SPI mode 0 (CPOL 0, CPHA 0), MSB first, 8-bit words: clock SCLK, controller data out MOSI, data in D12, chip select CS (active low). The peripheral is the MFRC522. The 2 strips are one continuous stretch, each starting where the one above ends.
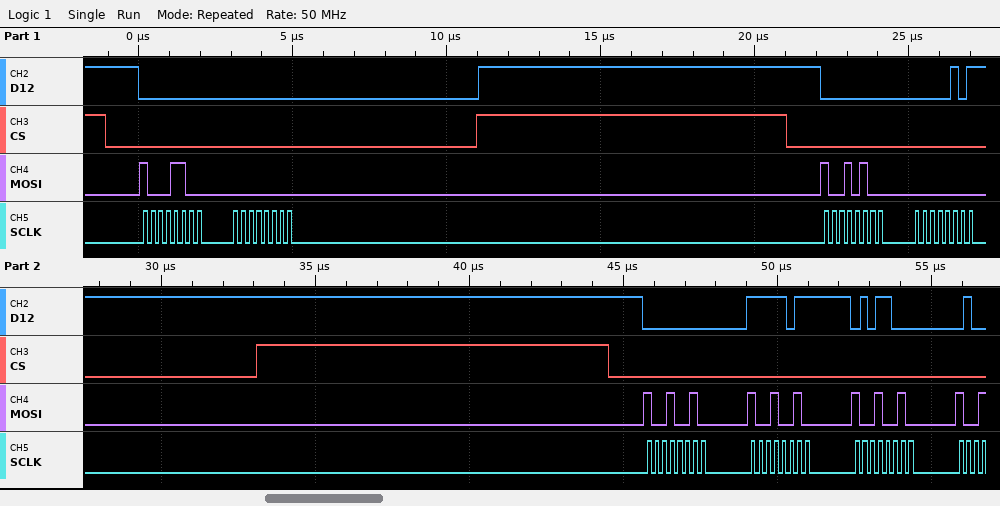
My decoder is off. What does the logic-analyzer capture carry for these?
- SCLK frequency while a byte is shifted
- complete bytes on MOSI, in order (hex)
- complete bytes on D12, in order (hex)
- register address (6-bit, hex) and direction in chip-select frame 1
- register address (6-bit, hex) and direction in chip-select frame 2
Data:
4 MHz
0x8C 0x00 0x94 0x00 0x92 0x92 0x92
0x00 0x00 0x00 0x05 0x00 0xFB 0x58
0x06 read
0x0A read
